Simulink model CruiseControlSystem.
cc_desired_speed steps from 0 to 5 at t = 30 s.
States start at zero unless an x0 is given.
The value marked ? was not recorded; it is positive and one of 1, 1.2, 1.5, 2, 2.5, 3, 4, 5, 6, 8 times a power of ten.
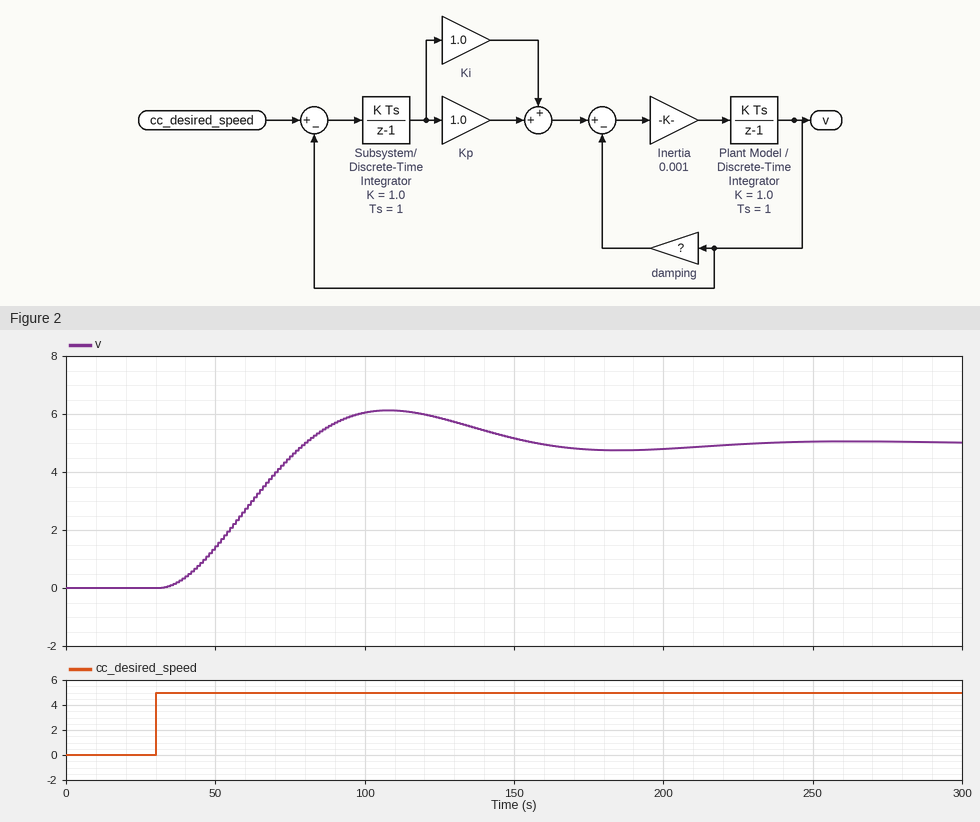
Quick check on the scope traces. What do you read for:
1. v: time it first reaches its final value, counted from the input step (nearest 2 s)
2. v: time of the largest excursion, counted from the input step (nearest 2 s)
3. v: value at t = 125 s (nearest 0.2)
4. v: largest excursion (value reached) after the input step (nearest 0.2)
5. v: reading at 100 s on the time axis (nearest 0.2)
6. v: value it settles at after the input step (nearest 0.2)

50 s
78 s
5.8
6.2
6.0
5.0
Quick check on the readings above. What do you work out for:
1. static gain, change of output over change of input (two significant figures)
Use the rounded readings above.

1.0
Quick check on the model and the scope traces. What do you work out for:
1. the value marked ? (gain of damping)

40
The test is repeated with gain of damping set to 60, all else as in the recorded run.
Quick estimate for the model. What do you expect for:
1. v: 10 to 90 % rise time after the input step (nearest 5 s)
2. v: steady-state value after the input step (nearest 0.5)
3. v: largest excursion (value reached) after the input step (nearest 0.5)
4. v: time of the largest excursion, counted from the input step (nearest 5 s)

45 s
5.0
5.5
90 s
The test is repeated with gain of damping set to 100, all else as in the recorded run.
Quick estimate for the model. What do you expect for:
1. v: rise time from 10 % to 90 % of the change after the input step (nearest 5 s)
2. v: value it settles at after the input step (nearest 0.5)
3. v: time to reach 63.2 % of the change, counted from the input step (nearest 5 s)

85 s
5.0
50 s
